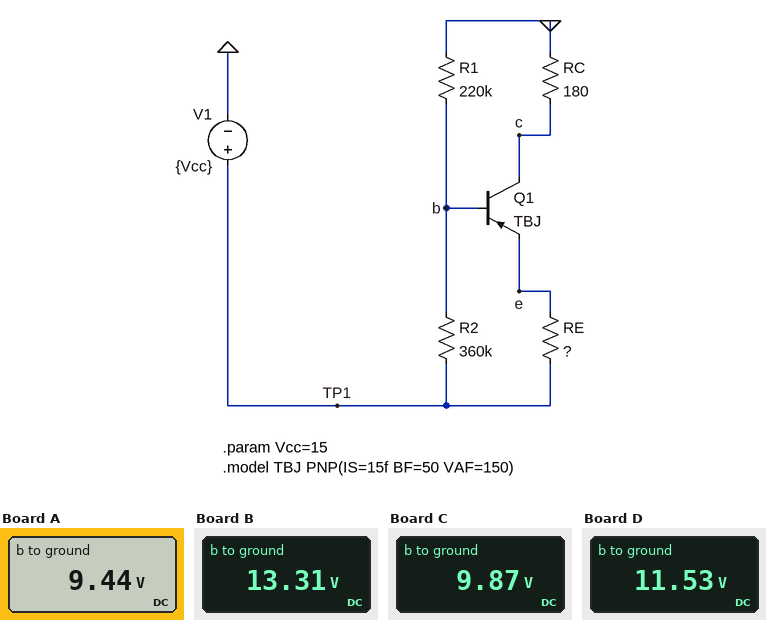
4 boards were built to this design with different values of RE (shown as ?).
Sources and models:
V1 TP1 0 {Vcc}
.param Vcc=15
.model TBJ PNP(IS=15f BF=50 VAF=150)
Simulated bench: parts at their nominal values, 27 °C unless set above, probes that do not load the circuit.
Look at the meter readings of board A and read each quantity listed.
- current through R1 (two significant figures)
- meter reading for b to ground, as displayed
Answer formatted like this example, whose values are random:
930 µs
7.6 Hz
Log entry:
43 µA
9.44 V
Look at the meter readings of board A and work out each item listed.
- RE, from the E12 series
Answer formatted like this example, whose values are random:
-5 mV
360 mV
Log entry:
3.3 kΩ
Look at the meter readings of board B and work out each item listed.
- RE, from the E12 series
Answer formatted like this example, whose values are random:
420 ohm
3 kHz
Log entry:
330 Ω
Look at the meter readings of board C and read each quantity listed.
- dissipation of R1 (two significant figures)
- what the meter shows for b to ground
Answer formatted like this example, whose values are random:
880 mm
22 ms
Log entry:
440 µW
9.87 V
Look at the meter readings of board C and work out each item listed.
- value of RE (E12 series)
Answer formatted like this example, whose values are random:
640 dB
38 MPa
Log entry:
2.7 kΩ
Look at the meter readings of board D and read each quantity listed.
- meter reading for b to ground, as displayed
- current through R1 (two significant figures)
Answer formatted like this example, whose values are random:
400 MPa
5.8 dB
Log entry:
11.53 V
52 µA
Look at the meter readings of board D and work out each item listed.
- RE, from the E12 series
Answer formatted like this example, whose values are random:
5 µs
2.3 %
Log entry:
1.2 kΩ
